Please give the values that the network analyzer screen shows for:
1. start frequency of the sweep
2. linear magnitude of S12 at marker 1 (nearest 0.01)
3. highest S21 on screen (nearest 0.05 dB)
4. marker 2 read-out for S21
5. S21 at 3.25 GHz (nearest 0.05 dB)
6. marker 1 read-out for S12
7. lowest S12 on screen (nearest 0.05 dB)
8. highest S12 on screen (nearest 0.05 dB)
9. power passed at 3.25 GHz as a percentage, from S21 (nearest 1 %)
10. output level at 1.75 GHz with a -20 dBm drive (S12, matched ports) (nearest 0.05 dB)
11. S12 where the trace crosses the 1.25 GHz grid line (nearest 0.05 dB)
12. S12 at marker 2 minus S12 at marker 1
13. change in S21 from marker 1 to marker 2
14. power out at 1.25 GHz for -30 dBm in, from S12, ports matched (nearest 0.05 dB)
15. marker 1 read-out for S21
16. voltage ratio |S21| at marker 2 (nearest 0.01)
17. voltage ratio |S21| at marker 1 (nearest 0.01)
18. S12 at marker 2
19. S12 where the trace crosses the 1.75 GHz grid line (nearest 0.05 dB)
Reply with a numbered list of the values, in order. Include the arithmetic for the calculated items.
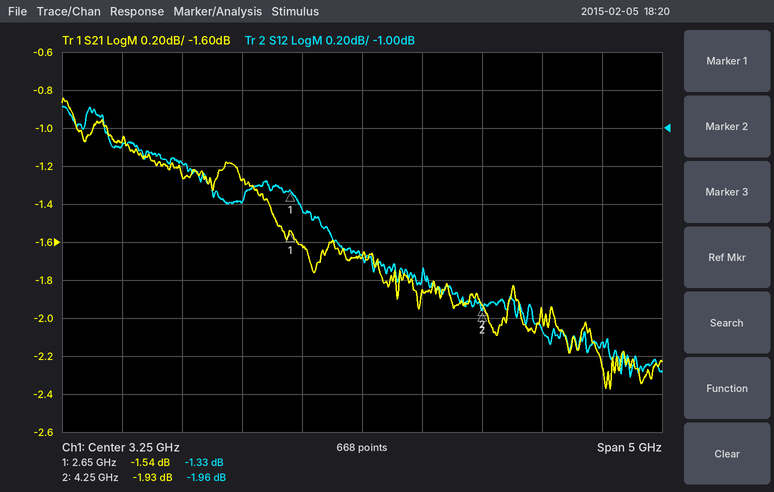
1. 750 MHz
2. 10^(-1.33/20) ≈ 0.86
3. -0.85 dB
4. -1.93 dB
5. -1.70 dB
6. -1.33 dB
7. -2.30 dB
8. -0.90 dB
9. 10^(-1.7/10) ≈ 68 %
10. -20 dBm + (-1.20 dB) = -21.20 dBm
11. -1.10 dB
12. -1.96 − (-1.33) = -0.63 dB
13. -1.93 − (-1.54) = -0.39 dB
14. -30 dBm + (-1.10 dB) = -31.10 dBm
15. -1.54 dB
16. 10^(-1.93/20) ≈ 0.80
17. 10^(-1.54/20) ≈ 0.84
18. -1.96 dB
19. -1.20 dB
